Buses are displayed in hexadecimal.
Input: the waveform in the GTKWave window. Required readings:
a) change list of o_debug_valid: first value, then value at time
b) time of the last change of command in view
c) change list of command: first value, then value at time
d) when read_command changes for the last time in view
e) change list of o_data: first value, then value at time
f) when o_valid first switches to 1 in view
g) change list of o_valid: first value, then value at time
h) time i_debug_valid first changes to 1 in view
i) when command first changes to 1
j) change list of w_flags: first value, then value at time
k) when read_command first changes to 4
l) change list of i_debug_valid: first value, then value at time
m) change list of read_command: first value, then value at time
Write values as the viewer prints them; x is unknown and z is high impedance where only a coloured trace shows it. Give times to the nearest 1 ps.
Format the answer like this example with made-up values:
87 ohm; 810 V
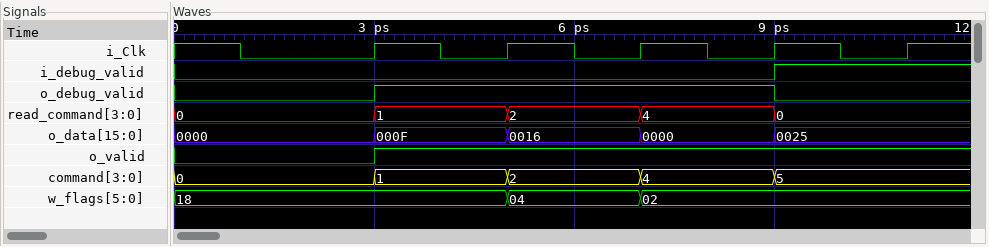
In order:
0, 1 at 3 ps, 0 at 9 ps; 9 ps; 0, 1 at 3 ps, 2 at 5 ps, 4 at 7 ps, 5 at 9 ps; 9 ps; 0000, 000F at 3 ps, 0016 at 5 ps, 0000 at 7 ps, 0025 at 9 ps; 3 ps; 0, 1 at 3 ps; 9 ps; 3 ps; 18, 04 at 5 ps, 02 at 7 ps; 7 ps; 0, 1 at 9 ps; 0, 1 at 3 ps, 2 at 5 ps, 4 at 7 ps, 0 at 9 ps
